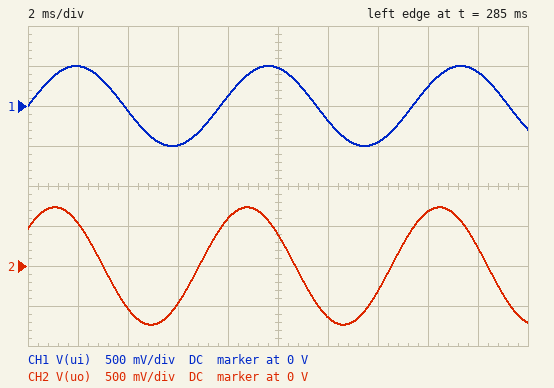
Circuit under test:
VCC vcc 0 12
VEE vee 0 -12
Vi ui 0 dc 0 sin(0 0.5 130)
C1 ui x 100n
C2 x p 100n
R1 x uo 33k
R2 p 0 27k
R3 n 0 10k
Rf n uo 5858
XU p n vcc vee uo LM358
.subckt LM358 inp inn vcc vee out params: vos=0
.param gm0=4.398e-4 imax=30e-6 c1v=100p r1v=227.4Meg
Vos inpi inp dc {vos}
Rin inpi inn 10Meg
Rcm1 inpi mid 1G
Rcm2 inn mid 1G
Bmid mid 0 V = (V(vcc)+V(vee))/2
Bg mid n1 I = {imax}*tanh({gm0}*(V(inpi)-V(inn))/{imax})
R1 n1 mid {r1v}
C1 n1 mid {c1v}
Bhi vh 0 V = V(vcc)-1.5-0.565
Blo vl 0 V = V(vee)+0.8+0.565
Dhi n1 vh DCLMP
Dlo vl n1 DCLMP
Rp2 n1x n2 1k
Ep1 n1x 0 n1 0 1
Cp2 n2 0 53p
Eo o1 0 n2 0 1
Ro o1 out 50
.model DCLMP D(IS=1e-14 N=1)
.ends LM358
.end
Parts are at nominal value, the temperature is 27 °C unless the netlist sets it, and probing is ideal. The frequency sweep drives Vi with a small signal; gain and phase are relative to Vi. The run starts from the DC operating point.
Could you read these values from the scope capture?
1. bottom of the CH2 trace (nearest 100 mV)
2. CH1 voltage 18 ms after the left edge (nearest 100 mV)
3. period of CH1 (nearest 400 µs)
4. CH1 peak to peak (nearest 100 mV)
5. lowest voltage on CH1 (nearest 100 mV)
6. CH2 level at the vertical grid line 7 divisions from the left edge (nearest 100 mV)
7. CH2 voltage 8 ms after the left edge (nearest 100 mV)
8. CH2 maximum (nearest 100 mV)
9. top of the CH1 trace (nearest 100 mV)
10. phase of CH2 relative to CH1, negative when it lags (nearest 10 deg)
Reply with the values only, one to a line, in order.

-700 mV
400 mV
7.6 ms
1.0 V
-500 mV
-300 mV
600 mV
700 mV
500 mV
40 deg
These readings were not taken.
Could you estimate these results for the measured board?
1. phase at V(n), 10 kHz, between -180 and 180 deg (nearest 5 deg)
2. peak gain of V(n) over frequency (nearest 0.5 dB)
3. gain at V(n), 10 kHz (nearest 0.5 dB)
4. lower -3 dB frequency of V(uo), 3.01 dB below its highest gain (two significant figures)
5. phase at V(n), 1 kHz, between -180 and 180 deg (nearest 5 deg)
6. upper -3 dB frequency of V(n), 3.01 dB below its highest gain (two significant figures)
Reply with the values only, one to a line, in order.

0 deg
0 dB
0 dB
65 Hz
5 deg
510 kHz
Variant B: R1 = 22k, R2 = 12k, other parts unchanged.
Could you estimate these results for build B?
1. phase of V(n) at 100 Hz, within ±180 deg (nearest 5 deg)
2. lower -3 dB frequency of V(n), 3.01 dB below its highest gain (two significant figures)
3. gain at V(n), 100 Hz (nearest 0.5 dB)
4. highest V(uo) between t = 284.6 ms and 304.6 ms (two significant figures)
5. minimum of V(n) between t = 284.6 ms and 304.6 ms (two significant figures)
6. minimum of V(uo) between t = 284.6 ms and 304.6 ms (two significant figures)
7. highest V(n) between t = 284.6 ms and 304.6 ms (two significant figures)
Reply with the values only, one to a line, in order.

90 deg
180 Hz
-7.0 dB
450 mV
-280 mV
-450 mV
280 mV
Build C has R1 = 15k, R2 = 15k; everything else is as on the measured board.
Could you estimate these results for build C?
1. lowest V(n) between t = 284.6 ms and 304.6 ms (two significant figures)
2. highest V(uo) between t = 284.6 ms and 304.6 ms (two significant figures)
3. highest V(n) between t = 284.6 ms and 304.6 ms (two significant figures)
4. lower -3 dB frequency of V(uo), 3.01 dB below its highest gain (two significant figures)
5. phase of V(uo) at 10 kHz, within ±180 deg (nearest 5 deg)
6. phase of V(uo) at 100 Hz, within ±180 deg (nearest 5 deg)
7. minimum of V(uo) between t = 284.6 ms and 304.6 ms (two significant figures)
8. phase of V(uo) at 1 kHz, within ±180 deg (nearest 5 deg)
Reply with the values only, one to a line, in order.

-420 mV
660 mV
420 mV
110 Hz
0 deg
95 deg
-660 mV
10 deg
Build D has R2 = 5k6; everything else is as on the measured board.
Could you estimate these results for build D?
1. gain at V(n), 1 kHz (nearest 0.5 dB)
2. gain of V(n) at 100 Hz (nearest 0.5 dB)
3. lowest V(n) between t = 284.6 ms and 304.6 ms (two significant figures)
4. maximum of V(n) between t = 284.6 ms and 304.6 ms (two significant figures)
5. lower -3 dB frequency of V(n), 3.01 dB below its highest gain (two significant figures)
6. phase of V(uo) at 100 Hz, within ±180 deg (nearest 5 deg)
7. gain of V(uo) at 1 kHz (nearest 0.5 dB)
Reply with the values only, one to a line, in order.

-1.0 dB
-14.5 dB
-120 mV
120 mV
510 Hz
95 deg
3.0 dB
